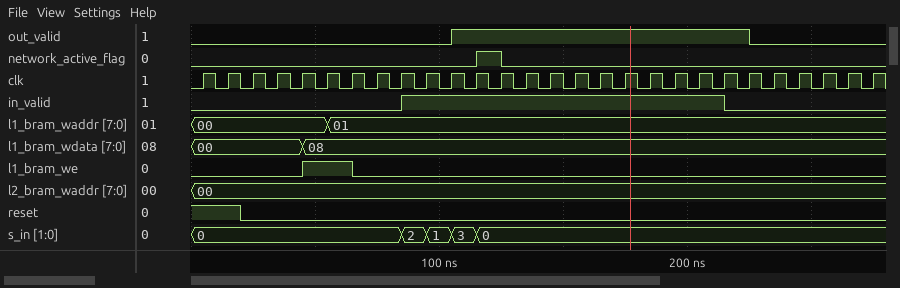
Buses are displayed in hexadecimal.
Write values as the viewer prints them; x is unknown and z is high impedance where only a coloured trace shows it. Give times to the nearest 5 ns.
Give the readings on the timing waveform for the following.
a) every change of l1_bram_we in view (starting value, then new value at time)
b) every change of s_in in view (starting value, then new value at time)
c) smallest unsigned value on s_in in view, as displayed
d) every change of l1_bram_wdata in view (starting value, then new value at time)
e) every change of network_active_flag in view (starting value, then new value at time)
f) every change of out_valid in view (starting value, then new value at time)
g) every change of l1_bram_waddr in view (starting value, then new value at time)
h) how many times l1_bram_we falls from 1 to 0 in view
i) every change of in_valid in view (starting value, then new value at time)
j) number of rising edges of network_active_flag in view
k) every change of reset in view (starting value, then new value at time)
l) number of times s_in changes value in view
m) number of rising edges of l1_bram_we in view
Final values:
0, 1 at 45 ns, 0 at 65 ns
0, 2 at 85 ns, 1 at 95 ns, 3 at 105 ns, 0 at 115 ns
0
00, 08 at 45 ns
0, 1 at 115 ns, 0 at 125 ns
0, 1 at 105 ns, 0 at 225 ns
00, 01 at 55 ns
1
0, 1 at 85 ns, 0 at 215 ns
1
1, 0 at 20 ns
4
1
